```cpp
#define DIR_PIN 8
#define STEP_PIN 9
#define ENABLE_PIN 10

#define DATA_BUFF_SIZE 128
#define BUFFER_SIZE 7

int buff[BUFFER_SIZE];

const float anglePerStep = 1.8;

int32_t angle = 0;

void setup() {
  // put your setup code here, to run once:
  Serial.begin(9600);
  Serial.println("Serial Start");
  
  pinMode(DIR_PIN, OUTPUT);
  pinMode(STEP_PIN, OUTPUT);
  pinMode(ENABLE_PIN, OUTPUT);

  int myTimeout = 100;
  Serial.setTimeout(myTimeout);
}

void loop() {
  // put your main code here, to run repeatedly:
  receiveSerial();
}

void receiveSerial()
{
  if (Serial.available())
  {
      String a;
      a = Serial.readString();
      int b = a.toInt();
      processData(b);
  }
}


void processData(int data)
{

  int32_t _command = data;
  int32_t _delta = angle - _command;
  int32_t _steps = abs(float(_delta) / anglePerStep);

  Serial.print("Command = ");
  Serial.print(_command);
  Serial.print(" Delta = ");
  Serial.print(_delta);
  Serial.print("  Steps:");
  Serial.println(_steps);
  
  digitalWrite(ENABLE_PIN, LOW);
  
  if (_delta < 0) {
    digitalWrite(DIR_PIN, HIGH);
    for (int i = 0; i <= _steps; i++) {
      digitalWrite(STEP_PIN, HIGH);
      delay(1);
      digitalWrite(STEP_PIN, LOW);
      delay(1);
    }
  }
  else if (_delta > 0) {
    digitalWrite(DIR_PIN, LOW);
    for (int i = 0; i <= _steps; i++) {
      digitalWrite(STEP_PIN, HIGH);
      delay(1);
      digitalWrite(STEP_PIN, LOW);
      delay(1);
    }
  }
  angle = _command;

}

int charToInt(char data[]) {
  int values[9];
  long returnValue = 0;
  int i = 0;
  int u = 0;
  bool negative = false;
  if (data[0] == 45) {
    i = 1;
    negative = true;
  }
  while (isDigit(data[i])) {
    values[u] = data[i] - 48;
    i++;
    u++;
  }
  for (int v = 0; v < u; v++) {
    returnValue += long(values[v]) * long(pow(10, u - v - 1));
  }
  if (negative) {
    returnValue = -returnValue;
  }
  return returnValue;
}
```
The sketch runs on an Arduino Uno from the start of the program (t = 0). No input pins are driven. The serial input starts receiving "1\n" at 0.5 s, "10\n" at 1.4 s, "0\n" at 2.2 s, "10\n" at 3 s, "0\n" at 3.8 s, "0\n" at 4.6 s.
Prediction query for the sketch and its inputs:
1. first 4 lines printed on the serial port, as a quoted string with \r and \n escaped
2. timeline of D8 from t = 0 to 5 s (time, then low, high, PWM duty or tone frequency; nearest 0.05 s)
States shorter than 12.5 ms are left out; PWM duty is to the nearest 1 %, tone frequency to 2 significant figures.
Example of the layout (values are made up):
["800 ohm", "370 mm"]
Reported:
["\"Serial Start\\r\\nCommand = 1 Delta = -1  Steps:0\\r\\nCommand = 10 Delta = -9  Steps:5\\r\\nCommand = 0 Delta = 10  Steps:5\\r\\n\"", "0 s low; 0.6 s high; 2.3 s low; 3.1 s high; 3.9 s low"]
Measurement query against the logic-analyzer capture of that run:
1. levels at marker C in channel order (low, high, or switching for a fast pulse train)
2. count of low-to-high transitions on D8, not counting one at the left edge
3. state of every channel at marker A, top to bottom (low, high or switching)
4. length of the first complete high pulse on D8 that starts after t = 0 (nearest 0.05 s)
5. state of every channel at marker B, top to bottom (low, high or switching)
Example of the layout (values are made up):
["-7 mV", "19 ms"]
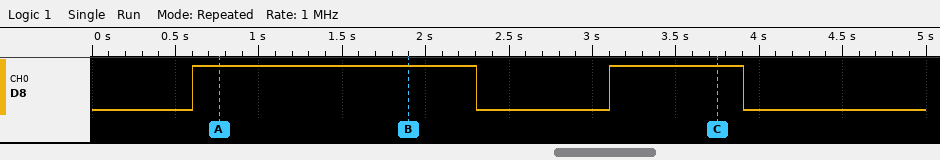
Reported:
["D8 high", "2", "D8 high", "1.70 s", "D8 high"]
